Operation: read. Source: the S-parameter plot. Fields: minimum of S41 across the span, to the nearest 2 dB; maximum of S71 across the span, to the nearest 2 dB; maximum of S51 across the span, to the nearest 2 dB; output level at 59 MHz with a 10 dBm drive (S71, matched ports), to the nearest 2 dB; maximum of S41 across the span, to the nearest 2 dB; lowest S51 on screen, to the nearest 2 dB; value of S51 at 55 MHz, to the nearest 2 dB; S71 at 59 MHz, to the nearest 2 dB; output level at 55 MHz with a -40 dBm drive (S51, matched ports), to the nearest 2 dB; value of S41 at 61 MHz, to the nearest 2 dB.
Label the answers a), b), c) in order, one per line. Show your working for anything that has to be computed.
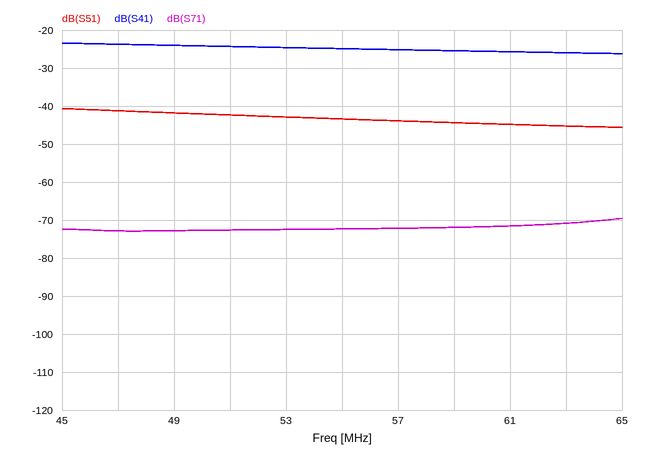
a) -26 dB
b) -70 dB
c) -40 dB
d) 10 dBm + (-72 dB) = -62 dBm
e) -24 dB
f) -46 dB
g) -44 dB
h) -72 dB
i) -40 dBm + (-44 dB) = -84 dBm
j) -26 dB
